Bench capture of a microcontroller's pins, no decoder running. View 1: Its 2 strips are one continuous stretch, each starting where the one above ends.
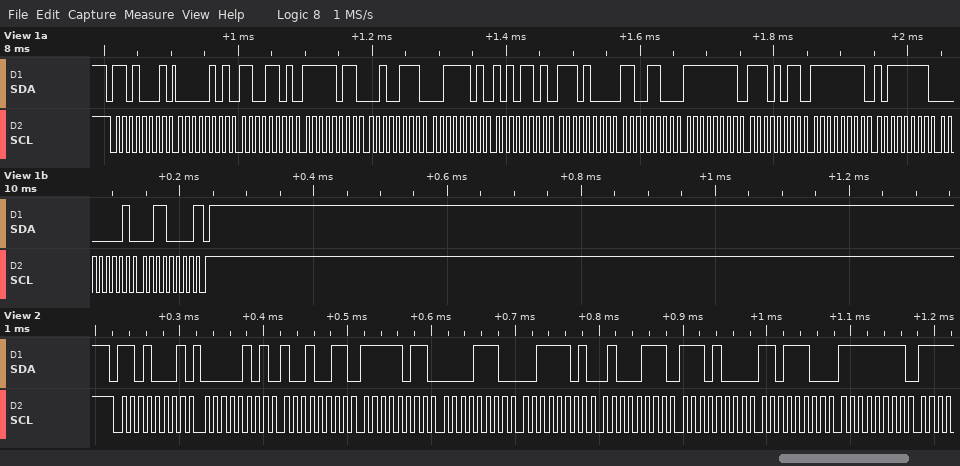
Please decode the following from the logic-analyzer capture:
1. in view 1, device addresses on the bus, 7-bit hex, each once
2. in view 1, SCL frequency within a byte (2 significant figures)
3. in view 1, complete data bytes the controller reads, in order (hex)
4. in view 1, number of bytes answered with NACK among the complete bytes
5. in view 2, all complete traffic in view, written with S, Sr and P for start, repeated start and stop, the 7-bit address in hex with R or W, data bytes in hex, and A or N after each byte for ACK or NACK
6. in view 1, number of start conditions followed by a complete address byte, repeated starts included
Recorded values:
0x68
100 kHz
05 CD FB 27 3D AD E8 CC FF EB FF BF 01 30
1
S 68R A 05 A 93 A FB A 0E A 3D A 47 A E8 A DC A FF A
1
